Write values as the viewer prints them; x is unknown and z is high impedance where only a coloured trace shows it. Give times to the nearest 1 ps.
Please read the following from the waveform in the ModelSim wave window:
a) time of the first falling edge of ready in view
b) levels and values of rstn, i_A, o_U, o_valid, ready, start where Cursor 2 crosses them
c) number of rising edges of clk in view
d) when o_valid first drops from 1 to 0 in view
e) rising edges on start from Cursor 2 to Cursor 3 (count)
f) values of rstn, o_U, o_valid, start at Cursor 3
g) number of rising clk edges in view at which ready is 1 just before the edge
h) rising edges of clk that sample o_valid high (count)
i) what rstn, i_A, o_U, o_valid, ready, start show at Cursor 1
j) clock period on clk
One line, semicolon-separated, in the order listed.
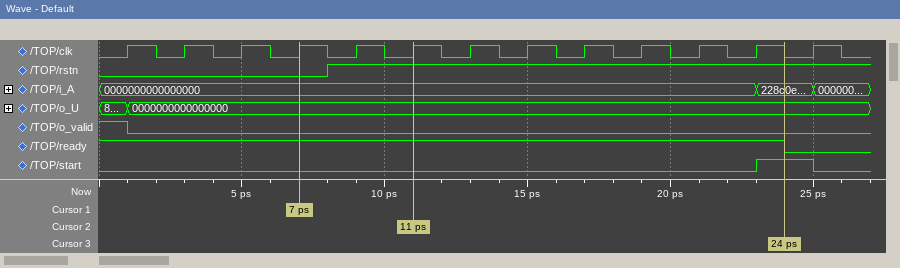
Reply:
24 ps; rstn=1, i_A=0000000000000000, o_U=0000000000000000, o_valid=0, ready=1, start=0; 13; 1 ps; 1; rstn=1, o_U=0000000000000000, o_valid=0, start=1; 12; 1; rstn=0, i_A=0000000000000000, o_U=0000000000000000, o_valid=0, ready=1, start=0; 2 ps
